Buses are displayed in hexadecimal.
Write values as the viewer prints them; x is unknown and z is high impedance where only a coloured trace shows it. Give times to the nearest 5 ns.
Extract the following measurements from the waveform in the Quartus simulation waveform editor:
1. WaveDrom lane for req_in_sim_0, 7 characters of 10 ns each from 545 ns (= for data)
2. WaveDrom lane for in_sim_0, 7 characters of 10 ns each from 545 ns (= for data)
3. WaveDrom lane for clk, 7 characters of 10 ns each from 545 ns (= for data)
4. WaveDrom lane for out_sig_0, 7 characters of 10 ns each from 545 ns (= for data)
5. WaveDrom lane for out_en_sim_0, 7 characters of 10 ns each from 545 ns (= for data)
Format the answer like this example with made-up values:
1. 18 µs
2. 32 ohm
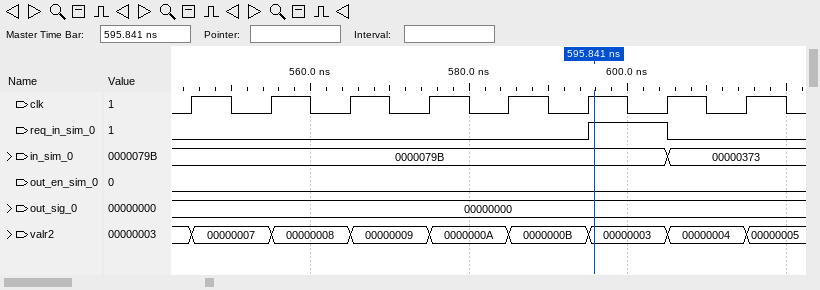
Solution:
1. {name: 'req_in_sim_0', wave: '0....10'}
2. {name: 'in_sim_0', wave: '=.....=', data: '0000079B 00000373'}
3. {name: 'clk', wave: 'p......'}
4. {name: 'out_sig_0', wave: '=......', data: '00000000'}
5. {name: 'out_en_sim_0', wave: '0......'}
